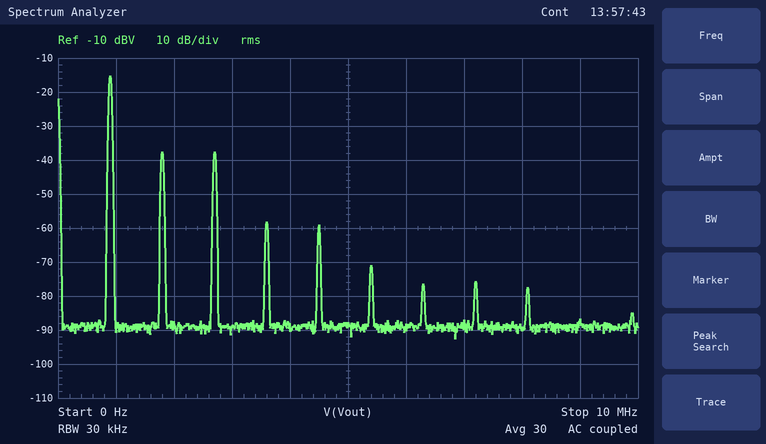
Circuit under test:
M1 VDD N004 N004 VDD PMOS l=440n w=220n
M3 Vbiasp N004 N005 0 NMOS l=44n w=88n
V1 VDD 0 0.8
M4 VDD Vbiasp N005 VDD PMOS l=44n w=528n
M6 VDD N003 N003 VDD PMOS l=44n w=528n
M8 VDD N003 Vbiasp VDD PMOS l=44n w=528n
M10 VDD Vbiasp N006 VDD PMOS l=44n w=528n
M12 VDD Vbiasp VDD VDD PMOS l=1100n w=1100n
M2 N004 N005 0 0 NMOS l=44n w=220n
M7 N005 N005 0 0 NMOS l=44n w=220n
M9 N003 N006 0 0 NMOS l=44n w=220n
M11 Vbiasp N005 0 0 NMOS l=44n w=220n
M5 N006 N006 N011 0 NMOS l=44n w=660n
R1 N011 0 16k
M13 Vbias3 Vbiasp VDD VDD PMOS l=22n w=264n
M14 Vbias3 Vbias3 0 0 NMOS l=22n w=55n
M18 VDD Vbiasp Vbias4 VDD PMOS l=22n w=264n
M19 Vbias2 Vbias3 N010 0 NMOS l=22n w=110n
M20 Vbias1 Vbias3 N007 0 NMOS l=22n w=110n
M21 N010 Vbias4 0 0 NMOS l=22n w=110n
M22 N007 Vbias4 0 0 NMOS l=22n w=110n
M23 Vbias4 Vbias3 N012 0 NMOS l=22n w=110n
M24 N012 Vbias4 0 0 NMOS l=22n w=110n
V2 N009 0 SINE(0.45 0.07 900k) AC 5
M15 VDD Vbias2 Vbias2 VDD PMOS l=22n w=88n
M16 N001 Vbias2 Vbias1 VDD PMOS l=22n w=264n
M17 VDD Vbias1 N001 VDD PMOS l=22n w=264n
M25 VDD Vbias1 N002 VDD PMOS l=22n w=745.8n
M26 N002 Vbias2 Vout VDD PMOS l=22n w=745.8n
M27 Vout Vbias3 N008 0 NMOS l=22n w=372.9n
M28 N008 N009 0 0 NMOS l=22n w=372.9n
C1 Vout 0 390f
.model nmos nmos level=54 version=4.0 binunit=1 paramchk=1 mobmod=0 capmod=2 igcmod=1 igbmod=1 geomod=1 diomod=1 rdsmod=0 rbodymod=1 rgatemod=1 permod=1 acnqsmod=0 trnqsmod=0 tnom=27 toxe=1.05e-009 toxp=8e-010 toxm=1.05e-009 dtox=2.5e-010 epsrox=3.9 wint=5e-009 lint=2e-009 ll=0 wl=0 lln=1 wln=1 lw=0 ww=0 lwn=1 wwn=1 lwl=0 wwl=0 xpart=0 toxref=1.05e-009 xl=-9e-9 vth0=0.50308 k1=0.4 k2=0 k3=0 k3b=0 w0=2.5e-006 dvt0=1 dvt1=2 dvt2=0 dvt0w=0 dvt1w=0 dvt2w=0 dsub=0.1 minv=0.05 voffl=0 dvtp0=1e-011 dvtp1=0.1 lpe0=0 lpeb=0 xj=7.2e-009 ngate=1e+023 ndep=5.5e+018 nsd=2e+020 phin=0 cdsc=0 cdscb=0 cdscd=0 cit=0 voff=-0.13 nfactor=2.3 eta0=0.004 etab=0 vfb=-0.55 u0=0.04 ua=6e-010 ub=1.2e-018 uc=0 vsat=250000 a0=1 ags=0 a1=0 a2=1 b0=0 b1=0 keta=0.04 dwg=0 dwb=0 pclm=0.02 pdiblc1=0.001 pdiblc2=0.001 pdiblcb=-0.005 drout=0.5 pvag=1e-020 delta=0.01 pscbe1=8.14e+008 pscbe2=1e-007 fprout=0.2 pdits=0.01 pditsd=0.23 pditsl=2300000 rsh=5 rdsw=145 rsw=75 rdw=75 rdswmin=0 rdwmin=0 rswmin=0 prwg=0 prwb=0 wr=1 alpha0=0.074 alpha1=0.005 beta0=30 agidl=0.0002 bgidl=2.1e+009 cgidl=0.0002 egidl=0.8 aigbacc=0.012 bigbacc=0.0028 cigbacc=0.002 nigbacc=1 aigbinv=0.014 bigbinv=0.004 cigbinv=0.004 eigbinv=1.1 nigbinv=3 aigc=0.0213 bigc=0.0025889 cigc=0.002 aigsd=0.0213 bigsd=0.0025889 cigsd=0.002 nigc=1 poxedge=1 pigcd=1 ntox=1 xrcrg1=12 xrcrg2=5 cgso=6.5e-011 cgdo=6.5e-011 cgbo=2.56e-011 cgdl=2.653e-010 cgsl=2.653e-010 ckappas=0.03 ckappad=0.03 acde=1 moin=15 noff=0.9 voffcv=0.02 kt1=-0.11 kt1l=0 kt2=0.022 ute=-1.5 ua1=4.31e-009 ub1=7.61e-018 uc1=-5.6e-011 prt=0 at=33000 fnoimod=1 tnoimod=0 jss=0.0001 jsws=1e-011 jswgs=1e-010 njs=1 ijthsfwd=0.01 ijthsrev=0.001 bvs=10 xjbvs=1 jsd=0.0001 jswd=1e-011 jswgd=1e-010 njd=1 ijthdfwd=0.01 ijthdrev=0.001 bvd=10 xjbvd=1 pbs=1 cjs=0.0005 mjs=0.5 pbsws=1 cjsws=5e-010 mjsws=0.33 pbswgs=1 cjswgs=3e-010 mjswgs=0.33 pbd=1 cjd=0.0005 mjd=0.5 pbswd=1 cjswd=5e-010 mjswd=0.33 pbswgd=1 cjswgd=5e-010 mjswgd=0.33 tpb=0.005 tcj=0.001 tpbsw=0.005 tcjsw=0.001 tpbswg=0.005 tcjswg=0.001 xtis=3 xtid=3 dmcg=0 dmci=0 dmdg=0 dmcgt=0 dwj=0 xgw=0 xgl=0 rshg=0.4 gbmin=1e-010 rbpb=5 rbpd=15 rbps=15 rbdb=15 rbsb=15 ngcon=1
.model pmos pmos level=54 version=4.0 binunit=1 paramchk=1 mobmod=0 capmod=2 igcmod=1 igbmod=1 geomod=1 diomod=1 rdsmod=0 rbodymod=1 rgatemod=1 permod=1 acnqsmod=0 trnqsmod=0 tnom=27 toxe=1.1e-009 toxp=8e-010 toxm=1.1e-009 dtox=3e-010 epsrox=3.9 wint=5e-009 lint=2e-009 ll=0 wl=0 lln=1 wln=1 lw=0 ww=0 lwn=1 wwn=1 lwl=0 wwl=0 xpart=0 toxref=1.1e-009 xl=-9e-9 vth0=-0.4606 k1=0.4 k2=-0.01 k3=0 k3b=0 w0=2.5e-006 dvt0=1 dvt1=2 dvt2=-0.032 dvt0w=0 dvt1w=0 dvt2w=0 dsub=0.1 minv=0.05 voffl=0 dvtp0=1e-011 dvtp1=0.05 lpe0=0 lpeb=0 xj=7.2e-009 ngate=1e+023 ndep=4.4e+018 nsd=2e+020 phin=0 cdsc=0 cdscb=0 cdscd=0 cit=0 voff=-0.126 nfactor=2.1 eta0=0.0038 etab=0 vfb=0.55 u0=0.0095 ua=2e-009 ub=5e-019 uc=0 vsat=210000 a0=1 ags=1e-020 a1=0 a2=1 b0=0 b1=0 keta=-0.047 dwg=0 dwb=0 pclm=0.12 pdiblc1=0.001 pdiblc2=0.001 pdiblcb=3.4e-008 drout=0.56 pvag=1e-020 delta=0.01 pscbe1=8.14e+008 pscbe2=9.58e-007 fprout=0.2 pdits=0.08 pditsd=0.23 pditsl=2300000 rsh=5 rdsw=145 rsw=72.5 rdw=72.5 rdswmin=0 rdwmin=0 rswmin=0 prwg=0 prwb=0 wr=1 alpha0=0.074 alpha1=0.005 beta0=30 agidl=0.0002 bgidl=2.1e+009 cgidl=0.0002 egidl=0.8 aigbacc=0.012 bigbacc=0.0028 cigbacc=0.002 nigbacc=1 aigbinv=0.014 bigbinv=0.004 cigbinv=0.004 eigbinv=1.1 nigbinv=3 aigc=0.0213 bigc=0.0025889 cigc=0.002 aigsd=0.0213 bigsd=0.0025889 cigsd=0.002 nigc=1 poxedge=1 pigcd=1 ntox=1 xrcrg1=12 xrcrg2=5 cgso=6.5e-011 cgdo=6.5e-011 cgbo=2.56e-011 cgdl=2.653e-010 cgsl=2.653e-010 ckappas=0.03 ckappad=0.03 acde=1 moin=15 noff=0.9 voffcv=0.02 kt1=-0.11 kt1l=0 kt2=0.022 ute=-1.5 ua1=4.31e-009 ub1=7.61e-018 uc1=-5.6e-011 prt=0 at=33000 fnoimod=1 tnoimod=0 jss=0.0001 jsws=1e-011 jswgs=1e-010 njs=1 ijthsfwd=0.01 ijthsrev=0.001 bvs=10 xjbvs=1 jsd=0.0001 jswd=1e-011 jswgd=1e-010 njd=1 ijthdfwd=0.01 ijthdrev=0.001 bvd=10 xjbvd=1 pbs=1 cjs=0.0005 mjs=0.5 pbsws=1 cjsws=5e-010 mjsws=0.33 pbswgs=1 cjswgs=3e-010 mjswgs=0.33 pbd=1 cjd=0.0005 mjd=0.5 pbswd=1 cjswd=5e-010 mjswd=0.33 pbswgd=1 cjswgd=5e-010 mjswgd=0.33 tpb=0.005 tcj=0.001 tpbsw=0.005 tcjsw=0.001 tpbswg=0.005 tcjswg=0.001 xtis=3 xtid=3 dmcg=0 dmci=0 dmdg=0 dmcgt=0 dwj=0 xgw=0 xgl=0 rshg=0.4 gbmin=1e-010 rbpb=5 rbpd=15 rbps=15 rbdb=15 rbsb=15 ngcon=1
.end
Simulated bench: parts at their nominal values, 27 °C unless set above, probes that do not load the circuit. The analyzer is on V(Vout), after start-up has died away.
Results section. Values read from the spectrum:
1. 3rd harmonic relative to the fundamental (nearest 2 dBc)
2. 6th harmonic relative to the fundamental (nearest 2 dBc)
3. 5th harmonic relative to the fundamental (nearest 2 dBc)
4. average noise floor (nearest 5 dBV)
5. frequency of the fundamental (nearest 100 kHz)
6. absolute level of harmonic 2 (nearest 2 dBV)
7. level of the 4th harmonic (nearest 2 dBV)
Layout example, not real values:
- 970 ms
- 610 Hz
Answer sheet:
- -22 dBc
- -56 dBc
- -44 dBc
- -90 dBV
- 900 kHz
- -38 dBV
- -58 dBV
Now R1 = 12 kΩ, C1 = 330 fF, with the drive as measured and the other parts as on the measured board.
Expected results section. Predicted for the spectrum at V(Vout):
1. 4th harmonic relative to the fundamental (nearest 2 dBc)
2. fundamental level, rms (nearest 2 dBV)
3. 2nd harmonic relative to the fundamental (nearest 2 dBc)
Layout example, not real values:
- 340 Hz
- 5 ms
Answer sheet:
- -36 dBc
- -16 dBV
- -18 dBc
